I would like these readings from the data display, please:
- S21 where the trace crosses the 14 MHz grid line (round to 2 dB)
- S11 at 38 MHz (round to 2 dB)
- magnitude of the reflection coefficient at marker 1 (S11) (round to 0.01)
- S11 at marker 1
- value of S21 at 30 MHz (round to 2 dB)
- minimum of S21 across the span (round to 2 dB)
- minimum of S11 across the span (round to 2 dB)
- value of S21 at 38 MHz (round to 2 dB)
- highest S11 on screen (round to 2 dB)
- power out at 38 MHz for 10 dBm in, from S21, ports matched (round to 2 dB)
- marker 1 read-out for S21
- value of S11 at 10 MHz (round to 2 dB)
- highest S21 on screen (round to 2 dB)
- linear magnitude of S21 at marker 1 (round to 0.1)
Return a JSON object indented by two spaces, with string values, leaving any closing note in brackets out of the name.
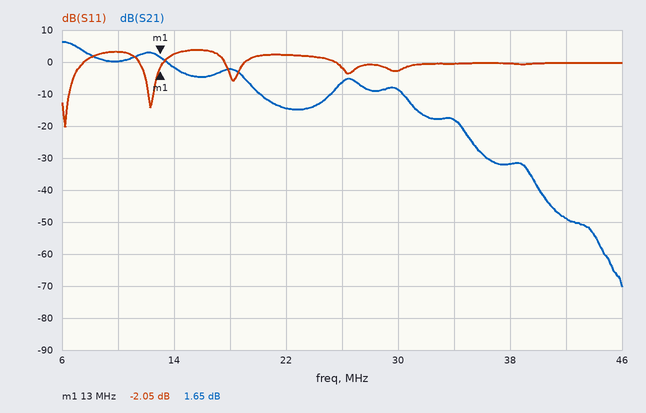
{
  "S21 where the trace crosses the 14 MHz grid line": "-2 dB",
  "S11 at 38 MHz": "0 dB",
  "magnitude of the reflection coefficient at marker 1 (S11)": "0.79",
  "S11 at marker 1": "-2.05 dB",
  "value of S21 at 30 MHz": "-8 dB",
  "minimum of S21 across the span": "-70 dB",
  "minimum of S11 across the span": "-20 dB",
  "value of S21 at 38 MHz": "-32 dB",
  "highest S11 on screen": "4 dB",
  "power out at 38 MHz for 10 dBm in, from S21, ports matched": "-22 dBm",
  "marker 1 read-out for S21": "1.65 dB",
  "value of S11 at 10 MHz": "4 dB",
  "highest S21 on screen": "6 dB",
  "linear magnitude of S21 at marker 1": "1.2"
}
